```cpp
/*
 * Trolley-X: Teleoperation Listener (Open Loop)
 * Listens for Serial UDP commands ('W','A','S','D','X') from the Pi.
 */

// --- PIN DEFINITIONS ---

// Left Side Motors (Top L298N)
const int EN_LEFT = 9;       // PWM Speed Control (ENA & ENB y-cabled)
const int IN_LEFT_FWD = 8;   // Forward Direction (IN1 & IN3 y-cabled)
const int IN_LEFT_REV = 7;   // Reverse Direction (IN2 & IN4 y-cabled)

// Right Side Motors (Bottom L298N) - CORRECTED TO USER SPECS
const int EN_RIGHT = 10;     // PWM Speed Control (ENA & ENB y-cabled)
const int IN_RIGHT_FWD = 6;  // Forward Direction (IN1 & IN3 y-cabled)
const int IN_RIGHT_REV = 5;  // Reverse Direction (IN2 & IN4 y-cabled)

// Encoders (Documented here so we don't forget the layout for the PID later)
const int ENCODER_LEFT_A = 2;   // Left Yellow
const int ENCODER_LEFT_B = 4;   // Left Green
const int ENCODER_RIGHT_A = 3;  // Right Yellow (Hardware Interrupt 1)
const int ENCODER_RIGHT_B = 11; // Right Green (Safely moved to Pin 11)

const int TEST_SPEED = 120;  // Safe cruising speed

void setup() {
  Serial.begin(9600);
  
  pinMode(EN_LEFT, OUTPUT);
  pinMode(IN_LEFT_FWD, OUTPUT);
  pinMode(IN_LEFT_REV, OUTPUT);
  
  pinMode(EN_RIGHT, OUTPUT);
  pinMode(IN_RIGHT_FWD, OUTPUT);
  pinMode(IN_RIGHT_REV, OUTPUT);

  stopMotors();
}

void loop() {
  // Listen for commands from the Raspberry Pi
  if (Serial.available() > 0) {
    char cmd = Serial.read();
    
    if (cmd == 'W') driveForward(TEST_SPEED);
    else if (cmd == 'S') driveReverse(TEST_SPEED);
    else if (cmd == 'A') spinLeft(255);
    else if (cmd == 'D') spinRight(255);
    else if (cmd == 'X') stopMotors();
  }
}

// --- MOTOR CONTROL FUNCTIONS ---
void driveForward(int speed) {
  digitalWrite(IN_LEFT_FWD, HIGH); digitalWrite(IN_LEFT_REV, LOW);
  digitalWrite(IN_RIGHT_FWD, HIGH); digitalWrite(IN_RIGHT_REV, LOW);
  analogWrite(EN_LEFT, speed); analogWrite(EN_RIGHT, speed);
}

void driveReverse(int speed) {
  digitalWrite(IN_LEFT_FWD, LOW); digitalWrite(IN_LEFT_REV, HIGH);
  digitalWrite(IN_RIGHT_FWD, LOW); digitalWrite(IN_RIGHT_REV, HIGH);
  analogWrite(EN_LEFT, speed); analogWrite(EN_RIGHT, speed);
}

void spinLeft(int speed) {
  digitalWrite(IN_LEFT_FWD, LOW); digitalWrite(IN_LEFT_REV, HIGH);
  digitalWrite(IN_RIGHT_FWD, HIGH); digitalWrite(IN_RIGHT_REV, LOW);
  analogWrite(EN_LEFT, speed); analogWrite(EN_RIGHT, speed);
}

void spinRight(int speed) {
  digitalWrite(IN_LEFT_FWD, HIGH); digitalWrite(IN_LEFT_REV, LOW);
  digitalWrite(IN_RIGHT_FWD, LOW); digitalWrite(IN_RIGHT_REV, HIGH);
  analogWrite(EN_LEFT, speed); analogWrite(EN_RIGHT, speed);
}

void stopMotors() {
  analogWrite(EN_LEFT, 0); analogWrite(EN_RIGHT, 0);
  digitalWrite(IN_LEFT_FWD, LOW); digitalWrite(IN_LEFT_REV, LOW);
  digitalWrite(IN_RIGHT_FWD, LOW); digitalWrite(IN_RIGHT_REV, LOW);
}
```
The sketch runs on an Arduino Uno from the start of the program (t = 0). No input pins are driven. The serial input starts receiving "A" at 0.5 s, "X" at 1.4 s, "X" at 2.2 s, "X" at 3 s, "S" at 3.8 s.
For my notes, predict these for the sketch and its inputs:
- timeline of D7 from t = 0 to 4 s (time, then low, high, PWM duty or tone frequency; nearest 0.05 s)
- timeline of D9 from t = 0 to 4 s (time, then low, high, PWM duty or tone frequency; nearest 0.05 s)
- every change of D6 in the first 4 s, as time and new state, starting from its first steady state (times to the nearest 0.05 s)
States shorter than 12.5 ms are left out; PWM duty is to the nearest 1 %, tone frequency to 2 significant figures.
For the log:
0 s low; 0.5 s high; 1.4 s low; 3.8 s high
0 s low; 0.5 s high; 1.4 s low; 3.8 s PWM 47 %
0 s low; 0.5 s high; 1.4 s low
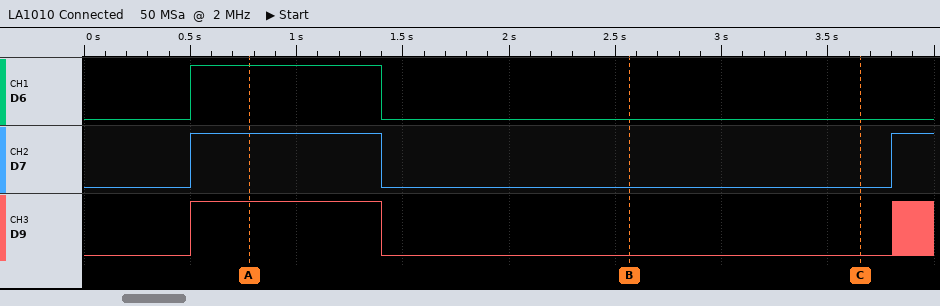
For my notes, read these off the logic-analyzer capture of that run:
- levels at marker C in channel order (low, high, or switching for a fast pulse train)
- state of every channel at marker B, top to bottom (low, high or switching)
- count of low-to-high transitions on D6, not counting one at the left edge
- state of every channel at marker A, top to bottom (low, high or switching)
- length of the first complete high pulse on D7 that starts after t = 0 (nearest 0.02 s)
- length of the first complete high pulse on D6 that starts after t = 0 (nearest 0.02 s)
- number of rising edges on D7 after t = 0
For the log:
D6 low, D7 low, D9 low
D6 low, D7 low, D9 low
1
D6 high, D7 high, D9 high
0.90 s
0.90 s
2
